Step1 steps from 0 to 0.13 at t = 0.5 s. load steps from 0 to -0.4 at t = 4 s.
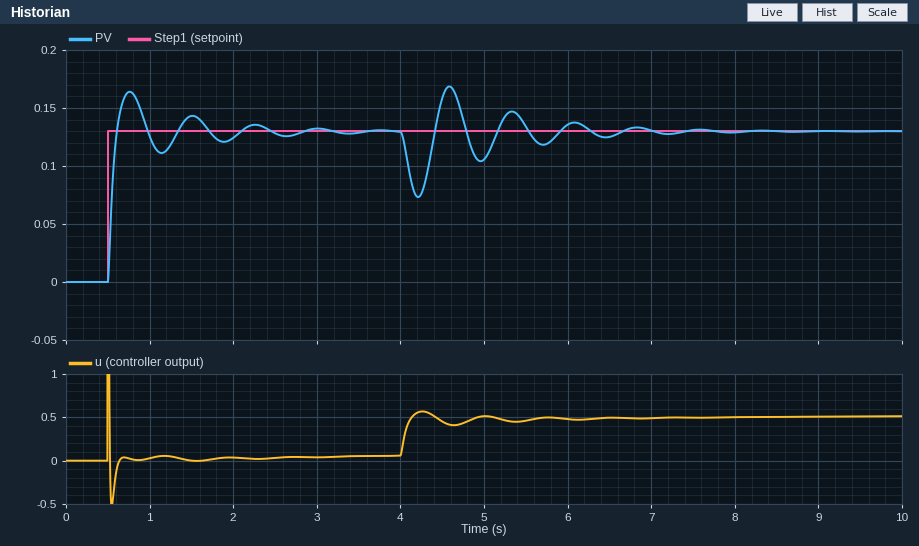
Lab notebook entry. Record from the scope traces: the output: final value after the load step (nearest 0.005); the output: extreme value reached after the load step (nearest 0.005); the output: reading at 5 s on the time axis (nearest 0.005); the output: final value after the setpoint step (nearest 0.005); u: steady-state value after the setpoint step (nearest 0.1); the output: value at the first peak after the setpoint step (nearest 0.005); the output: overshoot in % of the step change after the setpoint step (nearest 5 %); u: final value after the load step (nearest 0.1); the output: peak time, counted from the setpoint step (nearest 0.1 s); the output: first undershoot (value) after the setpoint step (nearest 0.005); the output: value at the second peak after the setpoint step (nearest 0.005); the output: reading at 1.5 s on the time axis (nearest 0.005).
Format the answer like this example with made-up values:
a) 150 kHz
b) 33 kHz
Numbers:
a) 0.130
b) 0.075
c) 0.105
d) 0.130
e) 0.1
f) 0.165
g) 25 %
h) 0.5
i) 0.3 s
j) 0.110
k) 0.145
l) 0.145
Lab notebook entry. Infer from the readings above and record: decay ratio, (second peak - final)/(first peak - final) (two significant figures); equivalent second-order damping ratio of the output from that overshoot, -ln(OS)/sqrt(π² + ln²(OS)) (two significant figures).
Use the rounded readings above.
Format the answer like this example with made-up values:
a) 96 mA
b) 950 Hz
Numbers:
a) 0.43
b) 0.40
